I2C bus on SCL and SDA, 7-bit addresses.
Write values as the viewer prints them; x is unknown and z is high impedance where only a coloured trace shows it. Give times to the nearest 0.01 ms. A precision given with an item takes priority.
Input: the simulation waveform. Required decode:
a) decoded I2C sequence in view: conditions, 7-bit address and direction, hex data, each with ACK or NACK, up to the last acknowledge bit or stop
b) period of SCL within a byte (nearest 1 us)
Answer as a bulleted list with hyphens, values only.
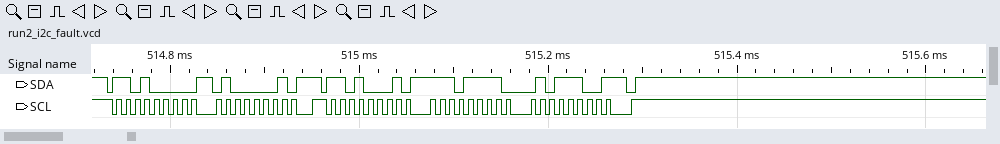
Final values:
- start, address 68 write ACK, 41 ACK, repeated start, address 68 read ACK, EF ACK, 5C NACK, stop
- 10 us
